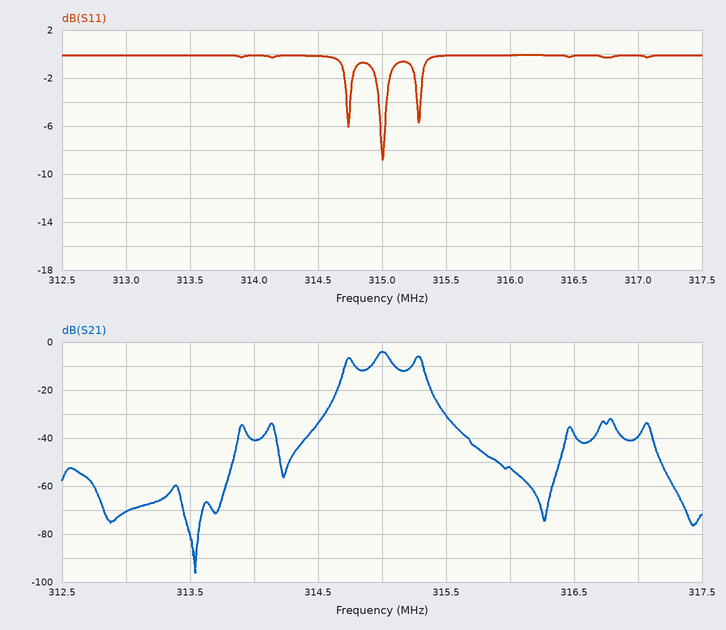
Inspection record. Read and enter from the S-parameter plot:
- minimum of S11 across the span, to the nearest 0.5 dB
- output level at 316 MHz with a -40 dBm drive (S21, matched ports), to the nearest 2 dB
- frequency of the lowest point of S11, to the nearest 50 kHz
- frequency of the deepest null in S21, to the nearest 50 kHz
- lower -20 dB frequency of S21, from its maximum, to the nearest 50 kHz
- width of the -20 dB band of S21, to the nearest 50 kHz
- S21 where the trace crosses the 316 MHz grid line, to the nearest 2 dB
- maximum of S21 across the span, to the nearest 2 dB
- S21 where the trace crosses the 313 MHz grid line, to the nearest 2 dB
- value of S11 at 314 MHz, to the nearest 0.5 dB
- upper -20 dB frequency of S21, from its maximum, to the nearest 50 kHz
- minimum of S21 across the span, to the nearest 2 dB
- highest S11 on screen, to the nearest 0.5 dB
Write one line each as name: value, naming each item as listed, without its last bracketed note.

minimum of S11 across the span, to the nearest 0.5 dB: -9.0 dB
output level at 316 MHz with a -40 dBm drive (S21, matched ports), to the nearest 2 dB: -92 dBm
frequency of the lowest point of S11, to the nearest 50 kHz: 315.00 MHz
frequency of the deepest null in S21, to the nearest 50 kHz: 313.55 MHz
lower -20 dB frequency of S21, from its maximum, to the nearest 50 kHz: 314.60 MHz
width of the -20 dB band of S21, to the nearest 50 kHz: 800 kHz
S21 where the trace crosses the 316 MHz grid line, to the nearest 2 dB: -52 dB
maximum of S21 across the span, to the nearest 2 dB: -4 dB
S21 where the trace crosses the 313 MHz grid line, to the nearest 2 dB: -70 dB
value of S11 at 314 MHz, to the nearest 0.5 dB: 0.0 dB
upper -20 dB frequency of S21, from its maximum, to the nearest 50 kHz: 315.40 MHz
minimum of S21 across the span, to the nearest 2 dB: -96 dB
highest S11 on screen, to the nearest 0.5 dB: 0.0 dB
